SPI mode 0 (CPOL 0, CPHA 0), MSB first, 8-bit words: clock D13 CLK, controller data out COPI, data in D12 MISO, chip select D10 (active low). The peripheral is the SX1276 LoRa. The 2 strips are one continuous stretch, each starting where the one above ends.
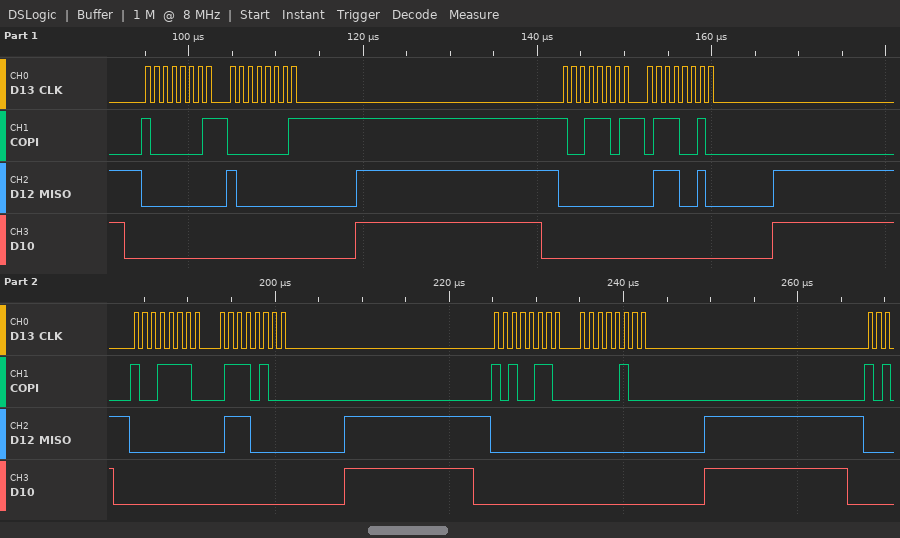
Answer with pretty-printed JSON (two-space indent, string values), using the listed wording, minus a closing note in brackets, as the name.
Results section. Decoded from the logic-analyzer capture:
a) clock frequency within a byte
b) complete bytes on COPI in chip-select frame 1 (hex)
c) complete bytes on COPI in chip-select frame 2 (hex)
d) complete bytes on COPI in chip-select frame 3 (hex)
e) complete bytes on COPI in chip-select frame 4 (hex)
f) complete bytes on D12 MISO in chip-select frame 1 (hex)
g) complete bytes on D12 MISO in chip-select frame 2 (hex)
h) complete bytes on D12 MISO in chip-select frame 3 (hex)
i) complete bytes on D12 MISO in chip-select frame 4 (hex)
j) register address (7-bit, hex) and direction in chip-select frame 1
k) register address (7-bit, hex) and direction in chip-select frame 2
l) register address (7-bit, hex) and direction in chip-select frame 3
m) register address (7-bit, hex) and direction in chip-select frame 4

{
  "clock frequency within a byte": "1 MHz",
  "complete bytes on COPI in chip-select frame 1": "0x81 0x01",
  "complete bytes on COPI in chip-select frame 2": "0x9D 0x72",
  "complete bytes on COPI in chip-select frame 3": "0x9E 0x74",
  "complete bytes on COPI in chip-select frame 4": "0xA6 0x04",
  "complete bytes on D12 MISO in chip-select frame 1": "0x00 0x80",
  "complete bytes on D12 MISO in chip-select frame 2": "0x00 0x72",
  "complete bytes on D12 MISO in chip-select frame 3": "0x00 0x70",
  "complete bytes on D12 MISO in chip-select frame 4": "0x00 0x00",
  "register address (7-bit, hex) and direction in chip-select frame 1": "0x01 write",
  "register address (7-bit, hex) and direction in chip-select frame 2": "0x1D write",
  "register address (7-bit, hex) and direction in chip-select frame 3": "0x1E write",
  "register address (7-bit, hex) and direction in chip-select frame 4": "0x26 write"
}
